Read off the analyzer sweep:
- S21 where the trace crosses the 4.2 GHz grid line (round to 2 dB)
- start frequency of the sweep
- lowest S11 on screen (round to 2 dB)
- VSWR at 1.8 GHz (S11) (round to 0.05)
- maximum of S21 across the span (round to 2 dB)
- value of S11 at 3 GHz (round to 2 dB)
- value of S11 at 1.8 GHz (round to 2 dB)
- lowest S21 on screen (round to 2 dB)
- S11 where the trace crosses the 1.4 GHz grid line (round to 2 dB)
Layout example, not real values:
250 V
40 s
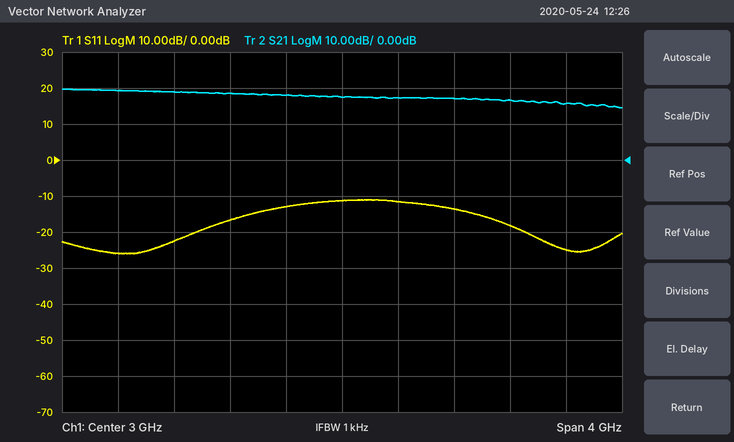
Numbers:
16 dB
1 GHz
-26 dB
1.15
20 dB
-12 dB
-22 dB
14 dB
-26 dB
